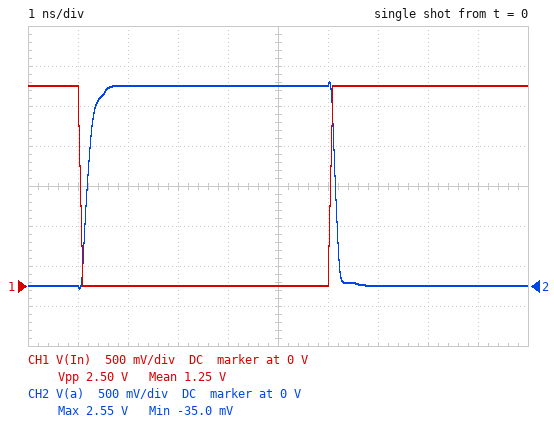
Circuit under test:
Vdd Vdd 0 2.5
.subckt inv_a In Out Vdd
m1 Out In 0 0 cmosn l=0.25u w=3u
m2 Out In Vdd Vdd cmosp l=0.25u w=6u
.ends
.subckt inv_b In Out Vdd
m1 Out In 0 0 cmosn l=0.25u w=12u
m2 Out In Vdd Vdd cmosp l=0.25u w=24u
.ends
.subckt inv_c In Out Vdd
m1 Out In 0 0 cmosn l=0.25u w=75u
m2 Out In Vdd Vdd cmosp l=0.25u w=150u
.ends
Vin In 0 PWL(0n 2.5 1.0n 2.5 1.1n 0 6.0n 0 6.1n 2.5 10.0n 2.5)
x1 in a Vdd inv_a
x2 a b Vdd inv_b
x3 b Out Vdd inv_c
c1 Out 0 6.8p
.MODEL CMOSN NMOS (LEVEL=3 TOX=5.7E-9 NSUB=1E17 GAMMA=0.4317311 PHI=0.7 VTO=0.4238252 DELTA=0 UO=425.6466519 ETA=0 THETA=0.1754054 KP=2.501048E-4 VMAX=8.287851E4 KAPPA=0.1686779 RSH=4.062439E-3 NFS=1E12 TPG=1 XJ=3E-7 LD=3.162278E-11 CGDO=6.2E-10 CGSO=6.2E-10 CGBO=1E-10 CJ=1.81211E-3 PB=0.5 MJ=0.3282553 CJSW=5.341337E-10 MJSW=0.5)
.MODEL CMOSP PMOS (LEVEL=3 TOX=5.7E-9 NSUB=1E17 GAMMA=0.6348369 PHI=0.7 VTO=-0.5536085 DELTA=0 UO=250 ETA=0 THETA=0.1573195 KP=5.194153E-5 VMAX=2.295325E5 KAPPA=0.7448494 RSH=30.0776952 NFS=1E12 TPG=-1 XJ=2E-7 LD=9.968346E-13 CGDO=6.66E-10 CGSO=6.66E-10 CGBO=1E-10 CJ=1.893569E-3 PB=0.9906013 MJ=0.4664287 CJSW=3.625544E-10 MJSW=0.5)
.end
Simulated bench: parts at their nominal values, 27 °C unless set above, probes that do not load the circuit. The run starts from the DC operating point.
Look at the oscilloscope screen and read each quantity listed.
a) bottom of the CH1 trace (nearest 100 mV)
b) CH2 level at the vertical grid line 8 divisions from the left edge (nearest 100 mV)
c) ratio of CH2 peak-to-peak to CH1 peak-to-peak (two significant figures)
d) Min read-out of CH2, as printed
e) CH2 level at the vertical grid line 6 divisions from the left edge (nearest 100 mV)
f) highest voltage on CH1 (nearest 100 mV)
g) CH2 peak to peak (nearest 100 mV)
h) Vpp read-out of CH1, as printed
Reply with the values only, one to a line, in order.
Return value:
0 V
0 V
1.0
-35.0 mV
2.5 V
2.5 V
2.6 V
2.50 V
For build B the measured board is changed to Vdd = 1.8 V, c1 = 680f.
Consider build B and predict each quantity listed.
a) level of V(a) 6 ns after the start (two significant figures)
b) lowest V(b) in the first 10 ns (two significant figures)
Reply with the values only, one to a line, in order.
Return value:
1.8 V
-25 mV
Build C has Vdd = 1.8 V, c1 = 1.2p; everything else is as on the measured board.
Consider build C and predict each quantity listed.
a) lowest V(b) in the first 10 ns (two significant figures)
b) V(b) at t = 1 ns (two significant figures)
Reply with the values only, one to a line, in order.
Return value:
-25 mV
1.8 V
